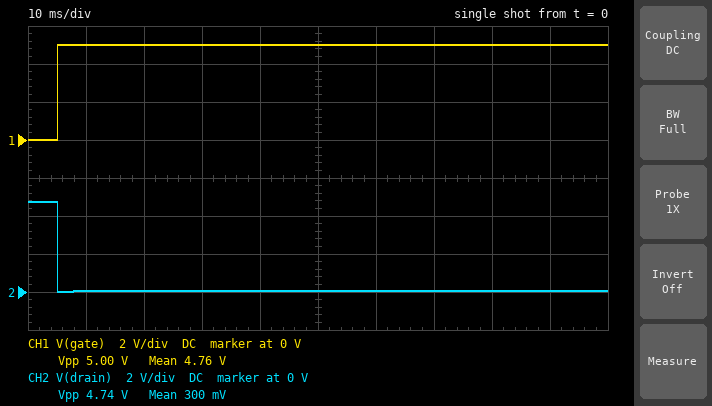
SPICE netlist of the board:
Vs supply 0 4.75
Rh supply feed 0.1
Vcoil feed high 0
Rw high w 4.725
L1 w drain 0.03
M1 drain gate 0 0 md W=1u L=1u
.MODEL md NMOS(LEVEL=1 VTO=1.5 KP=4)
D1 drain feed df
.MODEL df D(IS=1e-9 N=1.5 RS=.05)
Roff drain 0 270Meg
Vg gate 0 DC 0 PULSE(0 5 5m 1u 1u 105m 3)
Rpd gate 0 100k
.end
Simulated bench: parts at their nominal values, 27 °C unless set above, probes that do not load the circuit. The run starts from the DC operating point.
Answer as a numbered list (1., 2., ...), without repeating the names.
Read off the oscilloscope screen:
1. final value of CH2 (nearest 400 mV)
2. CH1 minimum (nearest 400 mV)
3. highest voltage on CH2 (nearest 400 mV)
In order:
1. 0 V
2. 0 V
3. 4.8 V
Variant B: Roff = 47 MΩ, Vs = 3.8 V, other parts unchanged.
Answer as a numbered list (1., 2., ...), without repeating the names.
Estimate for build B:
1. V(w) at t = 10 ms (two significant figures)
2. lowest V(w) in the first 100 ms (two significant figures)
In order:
1. 1.7 V
2. 56 mV
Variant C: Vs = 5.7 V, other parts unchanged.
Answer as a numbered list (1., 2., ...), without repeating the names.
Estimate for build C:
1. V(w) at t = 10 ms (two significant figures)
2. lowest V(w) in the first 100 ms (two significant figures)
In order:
1. 2.6 V
2. 84 mV
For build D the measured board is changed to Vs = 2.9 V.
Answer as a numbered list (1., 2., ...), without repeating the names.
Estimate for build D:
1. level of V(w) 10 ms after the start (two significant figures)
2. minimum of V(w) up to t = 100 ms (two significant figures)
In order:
1. 1.3 V
2. 43 mV
